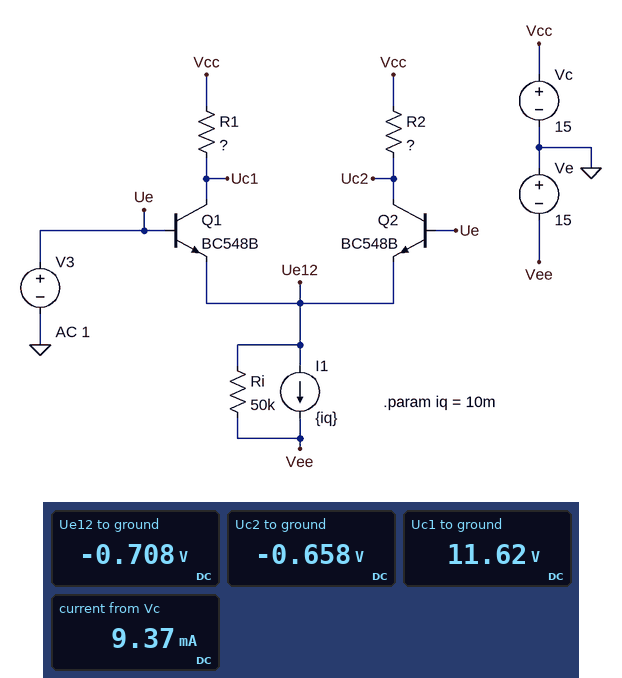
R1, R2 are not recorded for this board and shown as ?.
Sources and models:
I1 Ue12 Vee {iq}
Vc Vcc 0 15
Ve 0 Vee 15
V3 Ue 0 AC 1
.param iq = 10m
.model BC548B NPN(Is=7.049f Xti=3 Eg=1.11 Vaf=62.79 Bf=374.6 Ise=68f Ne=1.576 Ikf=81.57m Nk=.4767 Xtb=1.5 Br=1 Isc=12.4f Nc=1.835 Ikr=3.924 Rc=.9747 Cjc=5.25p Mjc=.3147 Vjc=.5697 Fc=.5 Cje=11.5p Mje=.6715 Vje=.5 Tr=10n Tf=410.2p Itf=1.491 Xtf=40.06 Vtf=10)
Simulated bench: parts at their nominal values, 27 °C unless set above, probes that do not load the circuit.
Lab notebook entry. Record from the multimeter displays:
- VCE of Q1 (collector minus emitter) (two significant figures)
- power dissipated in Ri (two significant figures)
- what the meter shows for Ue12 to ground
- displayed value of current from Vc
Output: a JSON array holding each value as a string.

["12 V", "4.1 mW", "-0.708 V", "9.37 mA"]
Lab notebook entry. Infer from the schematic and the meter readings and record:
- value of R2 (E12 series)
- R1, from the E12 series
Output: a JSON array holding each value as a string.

["4.7 kΩ", "560 Ω"]
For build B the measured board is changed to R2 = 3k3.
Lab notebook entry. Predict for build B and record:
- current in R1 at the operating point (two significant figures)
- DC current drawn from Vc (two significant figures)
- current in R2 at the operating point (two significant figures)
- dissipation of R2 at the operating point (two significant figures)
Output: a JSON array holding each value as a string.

["5.6 mA", "10 mA", "4.7 mA", "72 mW"]
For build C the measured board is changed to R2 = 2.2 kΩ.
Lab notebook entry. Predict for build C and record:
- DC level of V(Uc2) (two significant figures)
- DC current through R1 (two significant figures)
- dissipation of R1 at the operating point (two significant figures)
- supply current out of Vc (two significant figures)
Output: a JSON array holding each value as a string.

["4.3 V", "5.4 mA", "16 mW", "10 mA"]
